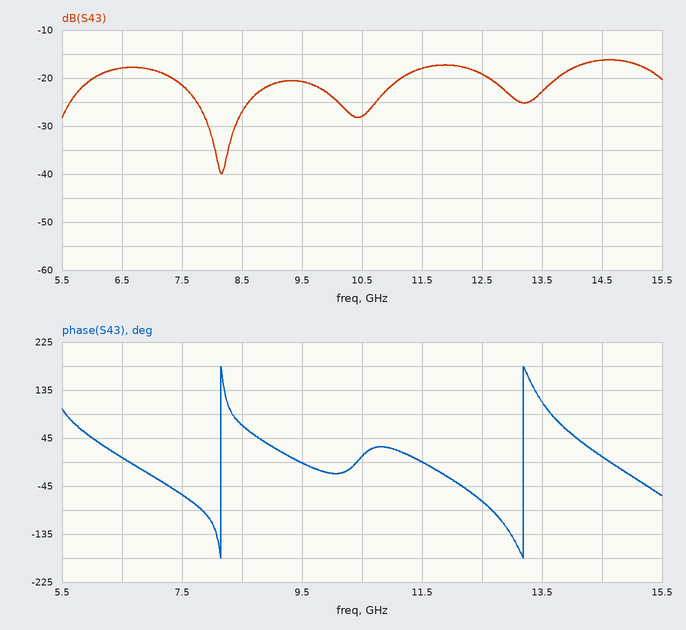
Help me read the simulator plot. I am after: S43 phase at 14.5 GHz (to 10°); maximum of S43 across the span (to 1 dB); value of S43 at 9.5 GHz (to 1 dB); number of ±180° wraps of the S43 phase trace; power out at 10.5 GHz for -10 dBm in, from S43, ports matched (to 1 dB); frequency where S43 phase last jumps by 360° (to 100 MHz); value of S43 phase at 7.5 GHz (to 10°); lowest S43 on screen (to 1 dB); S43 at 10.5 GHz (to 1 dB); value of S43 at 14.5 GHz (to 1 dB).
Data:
10°
-16 dB
-21 dB
2
-38 dBm
13.2 GHz
-60°
-40 dB
-28 dB
-16 dB
